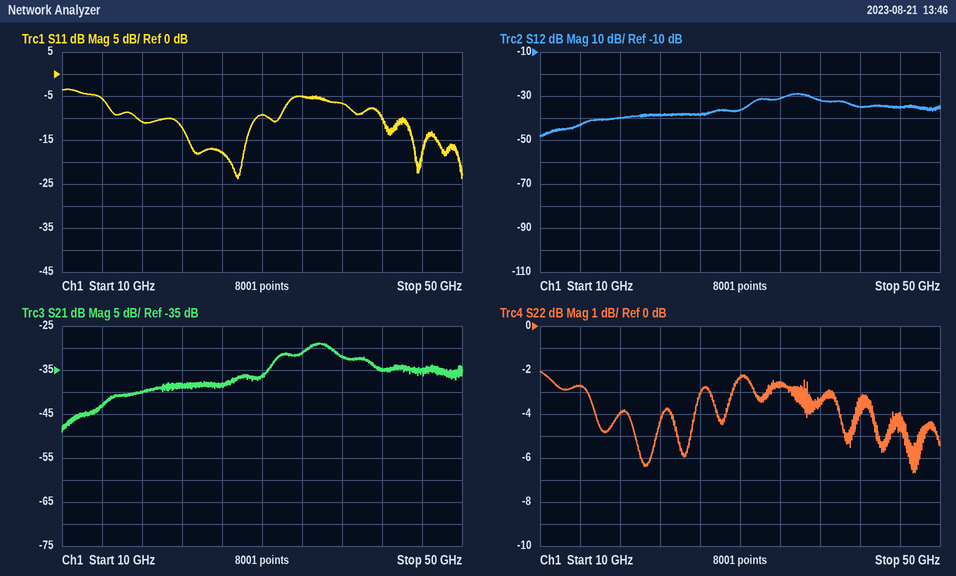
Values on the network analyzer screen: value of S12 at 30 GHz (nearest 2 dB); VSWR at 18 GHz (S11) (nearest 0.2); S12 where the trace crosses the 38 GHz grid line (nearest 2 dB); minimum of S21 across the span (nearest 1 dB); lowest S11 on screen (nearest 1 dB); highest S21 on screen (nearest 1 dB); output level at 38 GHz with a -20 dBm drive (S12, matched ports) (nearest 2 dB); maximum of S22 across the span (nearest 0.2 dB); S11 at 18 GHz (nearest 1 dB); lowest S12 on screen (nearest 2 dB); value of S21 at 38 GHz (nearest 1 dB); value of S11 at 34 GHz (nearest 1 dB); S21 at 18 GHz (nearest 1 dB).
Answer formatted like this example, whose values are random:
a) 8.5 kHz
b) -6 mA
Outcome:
a) -36 dB
b) 1.8
c) -32 dB
d) -49 dB
e) -24 dB
f) -29 dB
g) -52 dBm
h) -2.0 dB
i) -11 dB
j) -48 dB
k) -32 dB
l) -5 dB
m) -40 dB
